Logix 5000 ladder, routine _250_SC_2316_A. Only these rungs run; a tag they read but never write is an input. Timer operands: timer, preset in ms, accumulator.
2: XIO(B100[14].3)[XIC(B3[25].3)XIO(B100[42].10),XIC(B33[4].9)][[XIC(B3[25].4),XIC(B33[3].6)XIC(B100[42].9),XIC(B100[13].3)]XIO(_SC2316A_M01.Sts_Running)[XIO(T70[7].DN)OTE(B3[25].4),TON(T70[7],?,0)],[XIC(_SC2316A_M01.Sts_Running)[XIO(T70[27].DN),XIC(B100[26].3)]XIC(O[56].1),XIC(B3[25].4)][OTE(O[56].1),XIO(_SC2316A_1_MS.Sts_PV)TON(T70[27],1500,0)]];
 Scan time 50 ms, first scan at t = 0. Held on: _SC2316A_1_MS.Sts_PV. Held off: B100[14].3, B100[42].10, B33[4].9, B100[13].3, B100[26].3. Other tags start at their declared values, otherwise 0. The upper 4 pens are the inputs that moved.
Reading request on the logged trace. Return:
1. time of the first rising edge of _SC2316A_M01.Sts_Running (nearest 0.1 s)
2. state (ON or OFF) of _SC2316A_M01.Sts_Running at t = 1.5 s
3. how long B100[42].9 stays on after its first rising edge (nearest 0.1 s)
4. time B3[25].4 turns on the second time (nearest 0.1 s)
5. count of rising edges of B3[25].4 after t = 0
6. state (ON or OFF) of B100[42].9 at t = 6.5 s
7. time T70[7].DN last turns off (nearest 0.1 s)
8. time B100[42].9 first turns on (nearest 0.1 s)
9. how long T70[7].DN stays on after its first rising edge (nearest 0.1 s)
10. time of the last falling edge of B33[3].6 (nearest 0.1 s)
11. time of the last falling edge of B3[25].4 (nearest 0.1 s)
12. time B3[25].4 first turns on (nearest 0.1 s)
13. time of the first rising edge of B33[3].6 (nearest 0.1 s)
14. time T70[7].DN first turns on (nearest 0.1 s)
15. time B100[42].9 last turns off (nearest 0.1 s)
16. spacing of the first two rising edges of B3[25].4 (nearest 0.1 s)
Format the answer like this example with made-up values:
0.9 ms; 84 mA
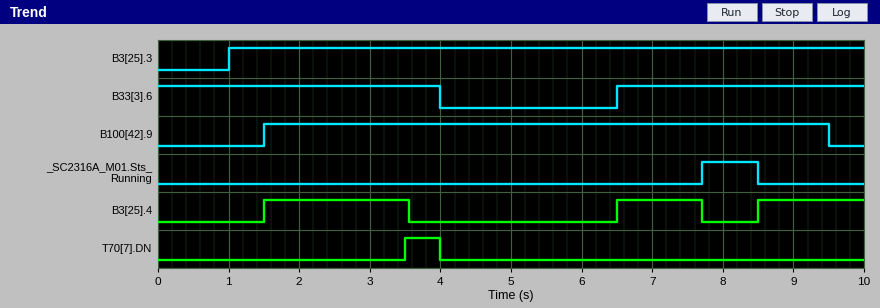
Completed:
7.7 s; OFF; 8.0 s; 6.5 s; 3; ON; 4.0 s; 1.5 s; 0.5 s; 4.0 s; 7.7 s; 1.5 s; 6.5 s; 3.5 s; 9.5 s; 5.0 s
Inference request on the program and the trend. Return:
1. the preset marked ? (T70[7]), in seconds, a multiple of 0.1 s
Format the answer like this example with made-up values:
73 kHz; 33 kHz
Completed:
2.0 s
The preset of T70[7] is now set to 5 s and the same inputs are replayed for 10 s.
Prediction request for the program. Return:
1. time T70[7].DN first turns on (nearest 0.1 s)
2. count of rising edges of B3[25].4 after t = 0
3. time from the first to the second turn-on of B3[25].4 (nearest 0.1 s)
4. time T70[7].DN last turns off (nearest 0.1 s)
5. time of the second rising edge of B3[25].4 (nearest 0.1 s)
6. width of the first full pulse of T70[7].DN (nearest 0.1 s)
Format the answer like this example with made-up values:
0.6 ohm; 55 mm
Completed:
6.5 s; 2; 7.0 s; 7.7 s; 8.5 s; 1.2 s
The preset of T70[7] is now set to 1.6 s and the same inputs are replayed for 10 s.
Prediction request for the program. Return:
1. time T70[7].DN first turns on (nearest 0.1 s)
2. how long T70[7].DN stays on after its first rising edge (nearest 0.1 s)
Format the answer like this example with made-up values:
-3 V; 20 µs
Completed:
3.1 s; 0.9 s
